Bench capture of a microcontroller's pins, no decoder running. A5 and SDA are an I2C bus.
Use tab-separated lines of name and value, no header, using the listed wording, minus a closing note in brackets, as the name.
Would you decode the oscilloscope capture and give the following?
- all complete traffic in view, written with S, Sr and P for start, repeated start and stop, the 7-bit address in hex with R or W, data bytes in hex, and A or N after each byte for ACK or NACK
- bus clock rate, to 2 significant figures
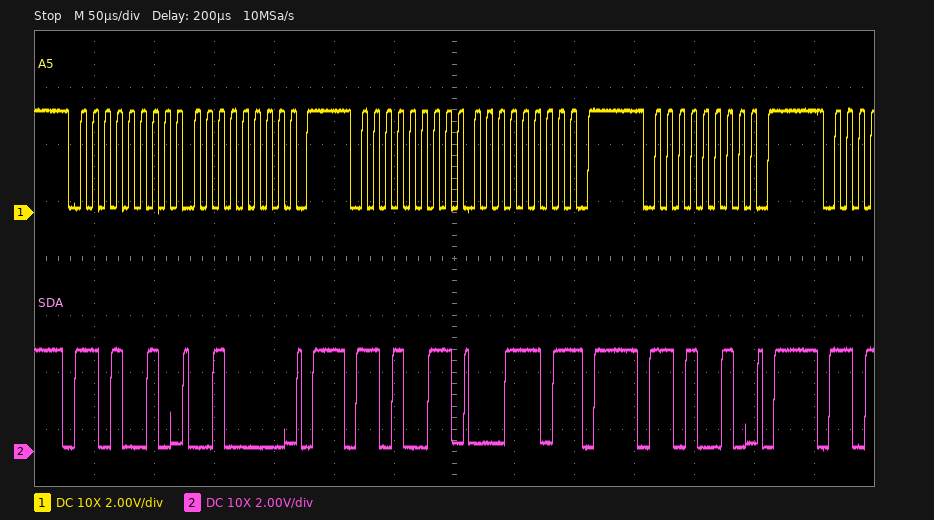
all complete traffic in view, written with S, Sr and P for start, repeated start and stop, the 7-bit address in hex with R or W, data bytes in hex, and A or N after each byte for ACK or NACK	S 69W A 20 A P S 69R A 1D N P S 69W A P
bus clock rate, to 2 significant figures	100 kHz
